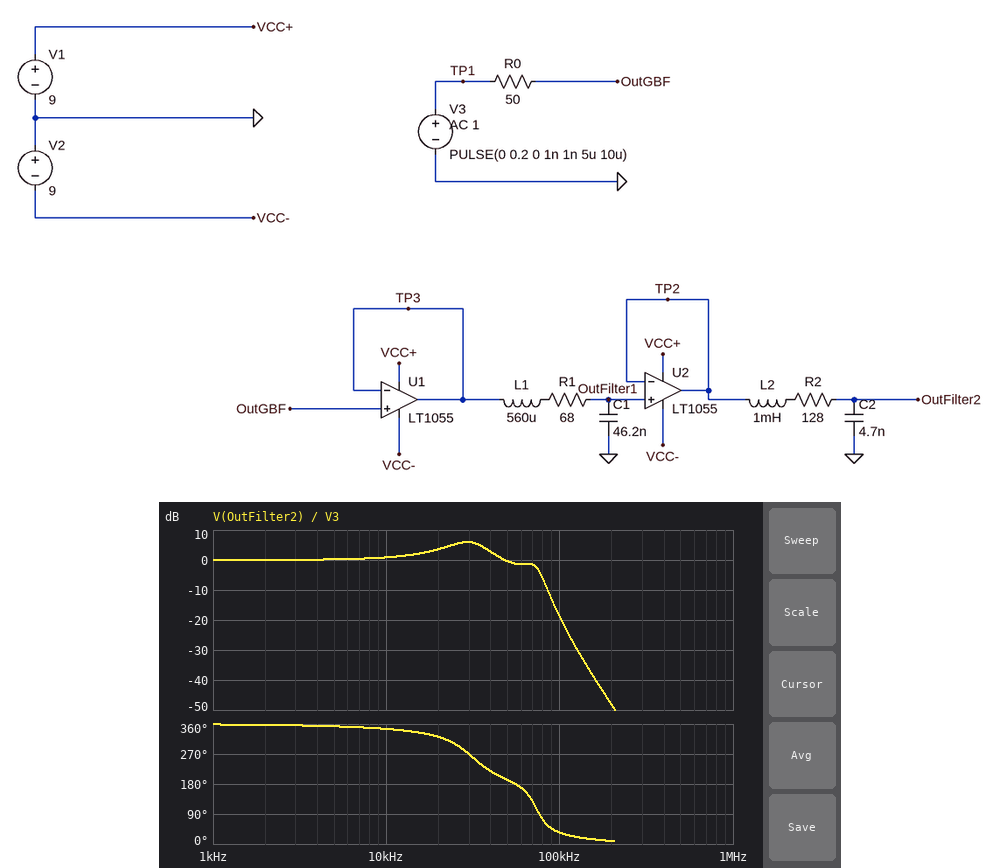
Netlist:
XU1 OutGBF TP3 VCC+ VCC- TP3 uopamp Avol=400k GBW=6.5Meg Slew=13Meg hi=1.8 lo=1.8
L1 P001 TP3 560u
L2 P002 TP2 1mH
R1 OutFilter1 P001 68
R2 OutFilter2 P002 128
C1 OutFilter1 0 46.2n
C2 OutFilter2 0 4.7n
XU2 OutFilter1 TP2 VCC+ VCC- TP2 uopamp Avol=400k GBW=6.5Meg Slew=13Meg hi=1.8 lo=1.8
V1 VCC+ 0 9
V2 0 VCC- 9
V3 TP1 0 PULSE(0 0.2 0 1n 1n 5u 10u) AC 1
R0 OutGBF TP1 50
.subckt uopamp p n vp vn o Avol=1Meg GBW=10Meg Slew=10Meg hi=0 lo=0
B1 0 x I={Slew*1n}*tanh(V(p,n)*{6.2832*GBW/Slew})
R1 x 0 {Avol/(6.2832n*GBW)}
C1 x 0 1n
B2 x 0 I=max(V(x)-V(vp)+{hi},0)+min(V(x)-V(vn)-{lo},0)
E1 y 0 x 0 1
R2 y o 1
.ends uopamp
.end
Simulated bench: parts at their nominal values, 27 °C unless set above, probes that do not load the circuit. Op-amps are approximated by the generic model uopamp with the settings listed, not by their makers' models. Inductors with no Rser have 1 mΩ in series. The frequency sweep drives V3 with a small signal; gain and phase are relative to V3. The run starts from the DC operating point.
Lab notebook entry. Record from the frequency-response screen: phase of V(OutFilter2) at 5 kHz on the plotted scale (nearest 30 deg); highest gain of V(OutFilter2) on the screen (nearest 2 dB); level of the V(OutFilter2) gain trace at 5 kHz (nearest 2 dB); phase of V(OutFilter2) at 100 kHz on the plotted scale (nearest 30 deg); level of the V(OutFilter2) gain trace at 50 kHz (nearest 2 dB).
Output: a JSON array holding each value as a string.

["360 deg", "6 dB", "0 dB", "30 deg", "0 dB"]
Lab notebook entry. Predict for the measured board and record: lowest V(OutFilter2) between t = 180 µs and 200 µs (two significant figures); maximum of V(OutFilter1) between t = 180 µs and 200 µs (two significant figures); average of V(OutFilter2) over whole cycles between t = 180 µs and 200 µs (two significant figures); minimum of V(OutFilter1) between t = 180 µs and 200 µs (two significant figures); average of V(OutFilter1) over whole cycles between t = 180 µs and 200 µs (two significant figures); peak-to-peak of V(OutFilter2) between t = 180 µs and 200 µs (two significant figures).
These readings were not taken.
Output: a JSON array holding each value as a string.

["86 mV", "110 mV", "100 mV", "87 mV", "100 mV", "29 mV"]
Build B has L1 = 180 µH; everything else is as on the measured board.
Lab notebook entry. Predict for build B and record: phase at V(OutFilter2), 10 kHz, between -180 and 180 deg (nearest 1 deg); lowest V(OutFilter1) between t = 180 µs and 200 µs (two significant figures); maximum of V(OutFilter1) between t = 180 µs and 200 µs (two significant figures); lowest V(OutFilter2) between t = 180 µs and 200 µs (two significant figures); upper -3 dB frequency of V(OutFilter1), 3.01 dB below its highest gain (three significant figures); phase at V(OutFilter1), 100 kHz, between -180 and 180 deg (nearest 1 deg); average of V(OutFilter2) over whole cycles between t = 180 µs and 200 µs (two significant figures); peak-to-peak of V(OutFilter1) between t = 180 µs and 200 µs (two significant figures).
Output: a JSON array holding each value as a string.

["-14 deg", "57 mV", "140 mV", "55 mV", "63.4 kHz", "-140 deg", "100 mV", "85 mV"]
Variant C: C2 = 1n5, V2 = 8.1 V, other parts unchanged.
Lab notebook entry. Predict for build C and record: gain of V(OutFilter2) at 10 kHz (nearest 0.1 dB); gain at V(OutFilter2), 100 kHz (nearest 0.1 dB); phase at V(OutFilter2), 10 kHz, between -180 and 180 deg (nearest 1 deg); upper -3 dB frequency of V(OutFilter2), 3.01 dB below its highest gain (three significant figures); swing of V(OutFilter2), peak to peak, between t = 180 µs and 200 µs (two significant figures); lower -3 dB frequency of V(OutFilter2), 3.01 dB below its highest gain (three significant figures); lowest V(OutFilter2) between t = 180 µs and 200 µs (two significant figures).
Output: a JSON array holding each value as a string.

["0.8 dB", "-12.1 dB", "-13 deg", "37.6 kHz", "64 mV", "16.0 kHz", "68 mV"]
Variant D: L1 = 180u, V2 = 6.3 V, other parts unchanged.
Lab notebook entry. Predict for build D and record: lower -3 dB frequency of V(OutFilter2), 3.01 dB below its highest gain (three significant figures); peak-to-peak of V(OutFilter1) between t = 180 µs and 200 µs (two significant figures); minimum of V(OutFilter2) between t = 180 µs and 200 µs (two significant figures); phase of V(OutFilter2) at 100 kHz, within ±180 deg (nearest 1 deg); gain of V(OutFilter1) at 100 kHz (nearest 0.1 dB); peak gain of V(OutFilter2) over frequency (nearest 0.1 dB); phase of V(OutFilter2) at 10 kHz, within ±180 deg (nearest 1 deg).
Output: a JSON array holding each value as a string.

["47.1 kHz", "85 mV", "55 mV", "63 deg", "-9.6 dB", "7.5 dB", "-14 deg"]
